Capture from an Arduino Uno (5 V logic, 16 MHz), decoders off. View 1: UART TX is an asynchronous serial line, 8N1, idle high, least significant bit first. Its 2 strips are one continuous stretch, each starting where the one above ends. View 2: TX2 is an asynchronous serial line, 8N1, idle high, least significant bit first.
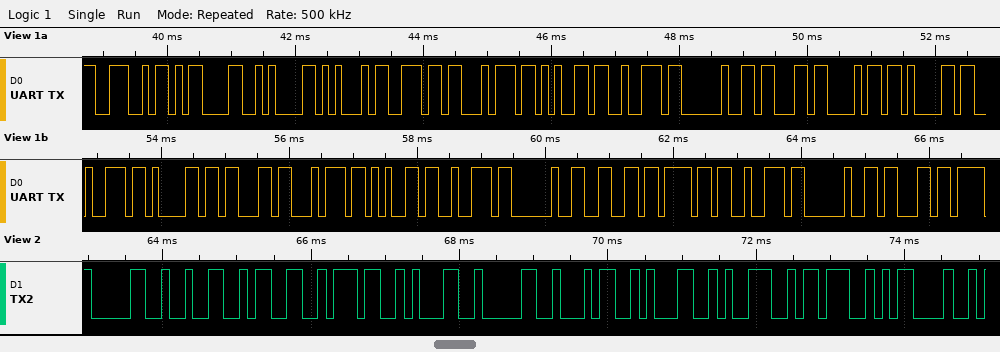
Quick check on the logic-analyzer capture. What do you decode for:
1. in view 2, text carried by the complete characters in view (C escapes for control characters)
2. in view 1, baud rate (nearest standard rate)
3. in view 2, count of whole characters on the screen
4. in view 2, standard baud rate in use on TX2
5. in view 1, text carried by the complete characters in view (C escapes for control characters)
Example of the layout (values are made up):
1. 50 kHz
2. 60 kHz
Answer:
1. "023710419;\r"
2. 9600 baud
3. 11
4. 9600 baud
5. "N\r\nEnter character for c"
